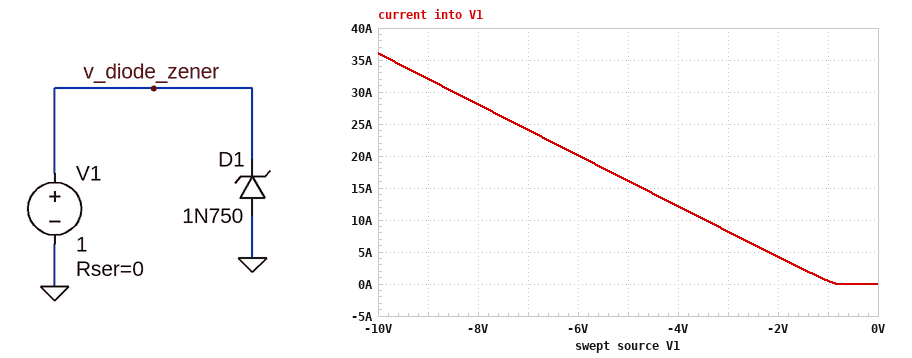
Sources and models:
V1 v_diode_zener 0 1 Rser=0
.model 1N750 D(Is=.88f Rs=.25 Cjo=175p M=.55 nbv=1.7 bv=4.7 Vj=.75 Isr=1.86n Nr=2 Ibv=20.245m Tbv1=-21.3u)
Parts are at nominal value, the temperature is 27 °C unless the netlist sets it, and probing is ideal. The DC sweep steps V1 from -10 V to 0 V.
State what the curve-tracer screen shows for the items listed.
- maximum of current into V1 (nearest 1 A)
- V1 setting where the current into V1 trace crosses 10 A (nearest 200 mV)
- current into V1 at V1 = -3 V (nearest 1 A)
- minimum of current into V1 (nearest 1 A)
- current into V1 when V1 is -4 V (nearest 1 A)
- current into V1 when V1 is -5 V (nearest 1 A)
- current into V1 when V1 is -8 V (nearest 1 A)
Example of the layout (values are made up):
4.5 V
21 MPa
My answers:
36 A
-3.4 V
8 A
0 A
12 A
16 A
28 A
